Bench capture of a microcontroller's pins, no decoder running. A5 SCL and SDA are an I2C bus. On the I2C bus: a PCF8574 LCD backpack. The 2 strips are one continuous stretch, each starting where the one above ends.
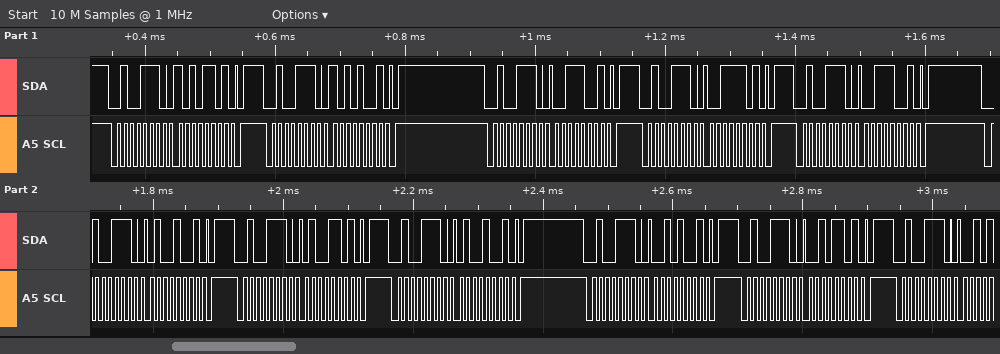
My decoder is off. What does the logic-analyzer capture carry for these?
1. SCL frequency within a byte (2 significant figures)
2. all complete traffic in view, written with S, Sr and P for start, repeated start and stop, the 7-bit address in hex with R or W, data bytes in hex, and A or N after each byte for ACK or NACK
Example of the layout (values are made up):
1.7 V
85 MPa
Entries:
100 kHz
S 27W A AD A P S 27W A A9 A P S 27W A 39 A P S 27W A 3D A P S 27W A 39 A P S 27W A 49 A P S 27W A 4D A P S 27W A 49 A P S 27W A 29 A P S 27W A 2D A P S 27W A
